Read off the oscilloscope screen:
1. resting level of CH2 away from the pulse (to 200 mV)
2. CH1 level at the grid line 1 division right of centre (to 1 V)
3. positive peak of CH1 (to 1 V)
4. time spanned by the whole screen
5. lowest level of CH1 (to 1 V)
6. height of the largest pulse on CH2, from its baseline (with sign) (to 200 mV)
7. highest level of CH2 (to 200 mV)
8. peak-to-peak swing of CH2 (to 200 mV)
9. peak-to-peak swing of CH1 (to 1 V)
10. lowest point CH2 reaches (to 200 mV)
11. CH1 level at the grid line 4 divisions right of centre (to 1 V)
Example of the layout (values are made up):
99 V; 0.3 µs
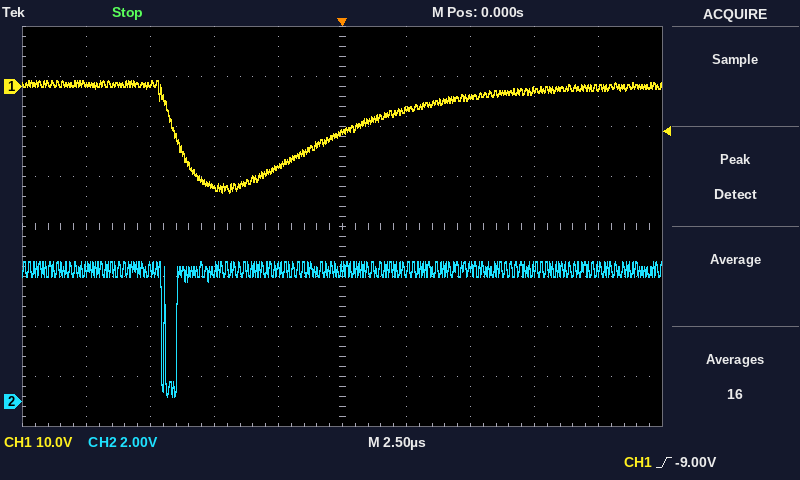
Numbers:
5.2 V; -5 V; 1 V; 25 µs; -21 V; -5.0 V; 5.6 V; 5.4 V; 22 V; 200 mV; 0 V
